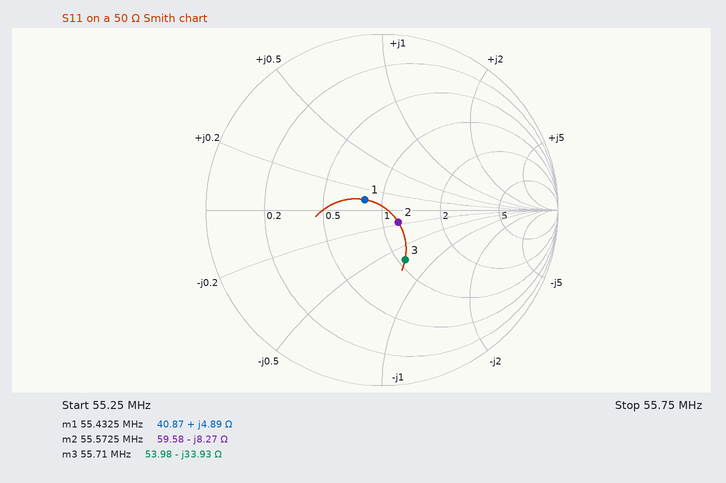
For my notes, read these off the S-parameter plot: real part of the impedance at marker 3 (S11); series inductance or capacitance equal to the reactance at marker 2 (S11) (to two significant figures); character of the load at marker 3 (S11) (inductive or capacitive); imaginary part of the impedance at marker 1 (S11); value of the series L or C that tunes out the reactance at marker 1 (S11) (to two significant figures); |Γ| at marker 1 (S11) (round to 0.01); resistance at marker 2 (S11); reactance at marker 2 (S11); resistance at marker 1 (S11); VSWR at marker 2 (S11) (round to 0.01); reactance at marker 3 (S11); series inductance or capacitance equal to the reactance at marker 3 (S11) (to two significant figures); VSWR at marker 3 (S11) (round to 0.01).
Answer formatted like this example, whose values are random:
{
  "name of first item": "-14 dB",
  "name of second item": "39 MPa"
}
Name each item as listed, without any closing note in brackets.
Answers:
{
  "real part of the impedance at marker 3": "53.98 Ω",
  "series inductance or capacitance equal to the reactance at marker 2 (S11)": "350 pF",
  "character of the load at marker 3 (S11)": "capacitive",
  "imaginary part of the impedance at marker 1": "+4.89 Ω",
  "value of the series L or C that tunes out the reactance at marker 1 (S11)": "590 pF",
  "|Γ| at marker 1 (S11)": "0.11",
  "resistance at marker 2": "59.58 Ω",
  "reactance at marker 2": "-8.27 Ω",
  "resistance at marker 1": "40.87 Ω",
  "VSWR at marker 2 (S11)": "1.26",
  "reactance at marker 3": "-33.93 Ω",
  "series inductance or capacitance equal to the reactance at marker 3 (S11)": "84 pF",
  "VSWR at marker 3 (S11)": "1.91"
}
